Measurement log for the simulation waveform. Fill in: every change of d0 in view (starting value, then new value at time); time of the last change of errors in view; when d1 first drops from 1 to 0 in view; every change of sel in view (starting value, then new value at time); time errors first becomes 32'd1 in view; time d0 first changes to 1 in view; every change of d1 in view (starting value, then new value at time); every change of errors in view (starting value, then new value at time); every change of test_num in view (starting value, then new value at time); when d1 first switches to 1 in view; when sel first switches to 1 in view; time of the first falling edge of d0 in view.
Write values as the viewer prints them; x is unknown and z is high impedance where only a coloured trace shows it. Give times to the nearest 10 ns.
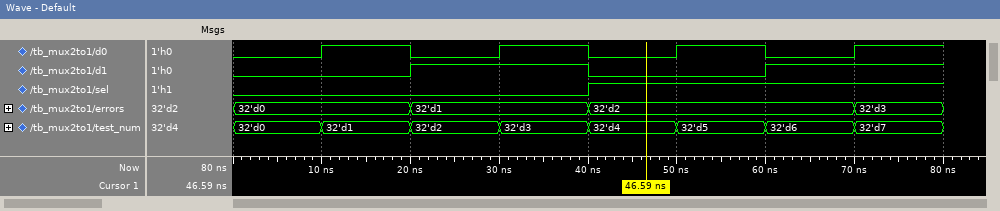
0, 1 at 10 ns, 0 at 20 ns, 1 at 30 ns, 0 at 40 ns, 1 at 50 ns, 0 at 60 ns, 1 at 70 ns
70 ns
40 ns
0, 1 at 40 ns
20 ns
10 ns
0, 1 at 20 ns, 0 at 40 ns, 1 at 60 ns
32'd0, 32'd1 at 20 ns, 32'd2 at 40 ns, 32'd3 at 70 ns
32'd0, 32'd1 at 10 ns, 32'd2 at 20 ns, 32'd3 at 30 ns, 32'd4 at 40 ns, 32'd5 at 50 ns, 32'd6 at 60 ns, 32'd7 at 70 ns
20 ns
40 ns
20 ns
